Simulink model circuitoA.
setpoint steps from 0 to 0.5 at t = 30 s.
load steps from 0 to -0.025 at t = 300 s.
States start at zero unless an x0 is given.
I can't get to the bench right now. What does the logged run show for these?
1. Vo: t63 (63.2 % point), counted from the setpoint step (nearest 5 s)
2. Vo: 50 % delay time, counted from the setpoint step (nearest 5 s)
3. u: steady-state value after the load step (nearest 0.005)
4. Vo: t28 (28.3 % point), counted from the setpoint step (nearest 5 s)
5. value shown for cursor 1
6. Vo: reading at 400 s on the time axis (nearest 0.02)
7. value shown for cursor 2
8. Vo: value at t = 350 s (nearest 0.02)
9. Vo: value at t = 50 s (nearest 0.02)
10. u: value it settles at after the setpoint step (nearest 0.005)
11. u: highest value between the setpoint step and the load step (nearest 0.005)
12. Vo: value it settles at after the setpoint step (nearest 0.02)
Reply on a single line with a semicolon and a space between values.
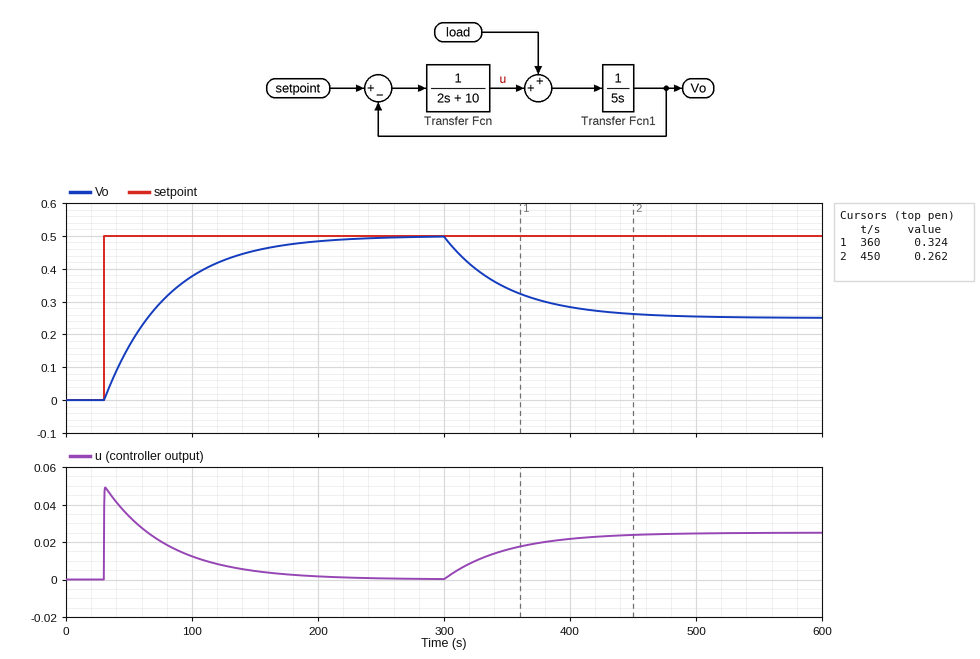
50 s; 35 s; 0.025; 15 s; 0.324; 0.28; 0.262; 0.34; 0.16; 0.000; 0.050; 0.50
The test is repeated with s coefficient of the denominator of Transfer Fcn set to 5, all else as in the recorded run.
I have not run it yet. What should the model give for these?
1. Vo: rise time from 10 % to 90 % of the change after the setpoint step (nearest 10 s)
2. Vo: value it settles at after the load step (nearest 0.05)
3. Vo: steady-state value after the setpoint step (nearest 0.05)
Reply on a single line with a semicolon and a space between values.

110 s; 0.25; 0.50
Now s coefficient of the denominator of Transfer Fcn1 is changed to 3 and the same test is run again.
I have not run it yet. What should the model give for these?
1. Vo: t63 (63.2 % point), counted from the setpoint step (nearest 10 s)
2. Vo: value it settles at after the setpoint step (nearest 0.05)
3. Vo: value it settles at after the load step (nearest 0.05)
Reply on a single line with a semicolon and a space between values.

30 s; 0.50; 0.25
